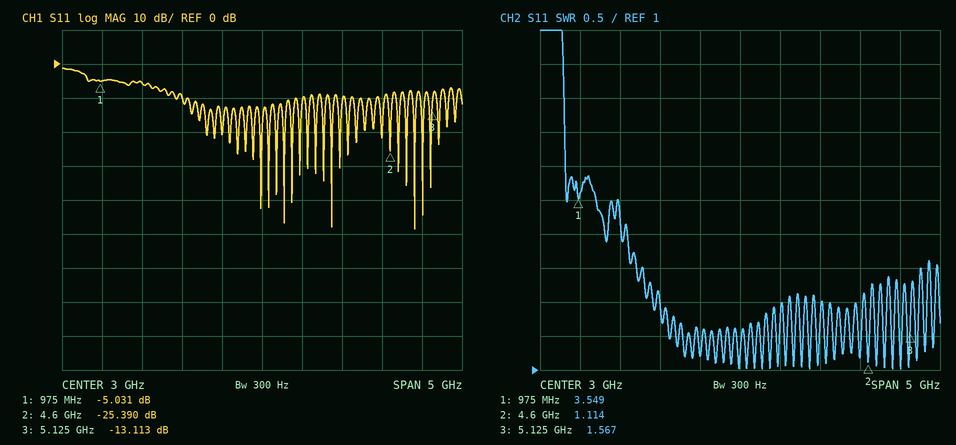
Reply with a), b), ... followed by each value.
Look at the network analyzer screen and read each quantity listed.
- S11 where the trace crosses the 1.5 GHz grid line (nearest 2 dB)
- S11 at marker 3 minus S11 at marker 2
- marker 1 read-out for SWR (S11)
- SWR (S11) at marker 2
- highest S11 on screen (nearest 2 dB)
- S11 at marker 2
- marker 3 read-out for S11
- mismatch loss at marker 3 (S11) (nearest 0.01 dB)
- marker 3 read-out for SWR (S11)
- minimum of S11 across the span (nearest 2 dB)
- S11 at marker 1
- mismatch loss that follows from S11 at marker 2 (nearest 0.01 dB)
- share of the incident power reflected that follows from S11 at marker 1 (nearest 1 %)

a) -6 dB
b) 12.277 dB
c) 3.549
d) 1.114
e) -2 dB
f) -25.390 dB
g) -13.113 dB
h) 0.22 dB
i) 1.567
j) -48 dB
k) -5.031 dB
l) 0.01 dB
m) 31 %
